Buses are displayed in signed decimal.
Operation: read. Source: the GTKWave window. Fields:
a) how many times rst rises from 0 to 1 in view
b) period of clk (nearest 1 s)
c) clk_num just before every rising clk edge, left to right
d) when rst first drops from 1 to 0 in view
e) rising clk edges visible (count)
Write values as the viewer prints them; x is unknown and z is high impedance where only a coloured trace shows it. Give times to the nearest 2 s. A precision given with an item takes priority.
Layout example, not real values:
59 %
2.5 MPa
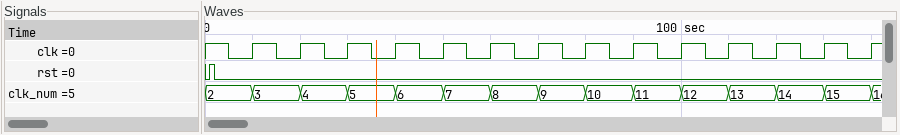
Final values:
1
10 s
2, 3, 4, 5, 6, 7, 8, 9, 10, 11, 12, 13, 14, 15
2 s
14
